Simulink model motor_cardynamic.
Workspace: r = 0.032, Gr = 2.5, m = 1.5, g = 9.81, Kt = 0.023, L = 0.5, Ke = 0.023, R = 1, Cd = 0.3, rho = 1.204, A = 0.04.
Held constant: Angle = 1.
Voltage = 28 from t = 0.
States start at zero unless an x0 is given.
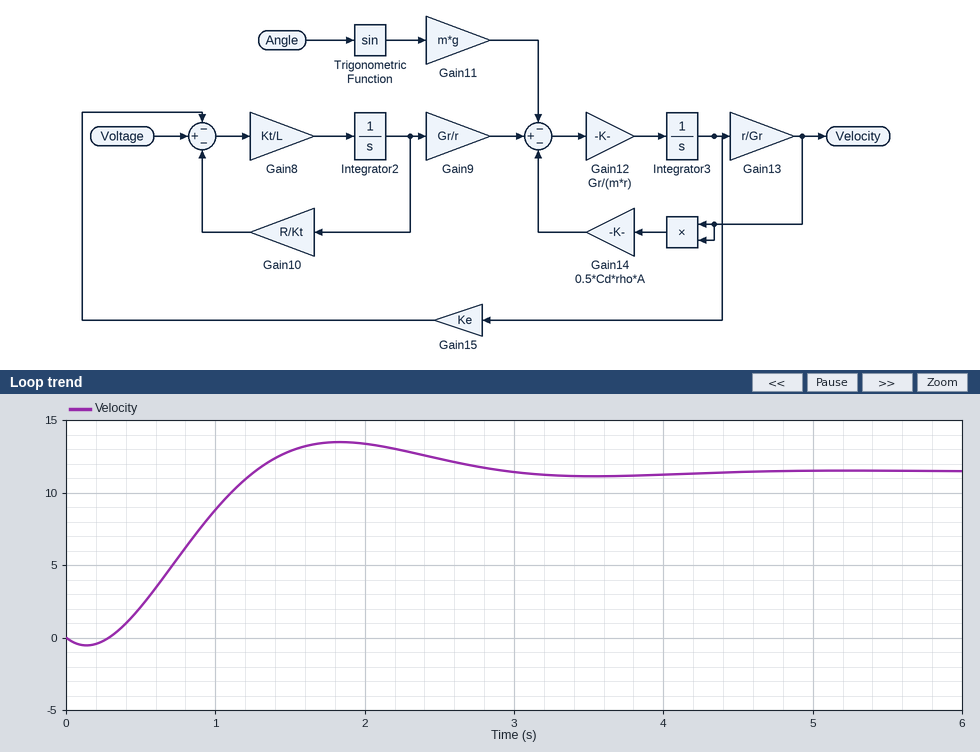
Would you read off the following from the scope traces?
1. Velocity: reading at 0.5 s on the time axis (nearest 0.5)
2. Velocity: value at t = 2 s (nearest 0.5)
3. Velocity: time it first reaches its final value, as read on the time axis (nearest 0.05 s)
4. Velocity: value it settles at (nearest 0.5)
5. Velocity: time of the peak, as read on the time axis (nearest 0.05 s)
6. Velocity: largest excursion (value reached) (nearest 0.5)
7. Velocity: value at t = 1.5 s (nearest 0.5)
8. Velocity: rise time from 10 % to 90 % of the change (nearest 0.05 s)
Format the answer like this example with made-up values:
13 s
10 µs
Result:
2.0
13.5
1.25 s
11.5
1.85 s
13.5
13.0
0.70 s
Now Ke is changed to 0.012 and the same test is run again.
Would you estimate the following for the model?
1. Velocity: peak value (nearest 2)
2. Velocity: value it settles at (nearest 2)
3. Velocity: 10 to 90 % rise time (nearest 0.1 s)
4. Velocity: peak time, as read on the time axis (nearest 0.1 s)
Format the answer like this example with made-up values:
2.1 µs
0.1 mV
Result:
22
20
1.2 s
2.8 s
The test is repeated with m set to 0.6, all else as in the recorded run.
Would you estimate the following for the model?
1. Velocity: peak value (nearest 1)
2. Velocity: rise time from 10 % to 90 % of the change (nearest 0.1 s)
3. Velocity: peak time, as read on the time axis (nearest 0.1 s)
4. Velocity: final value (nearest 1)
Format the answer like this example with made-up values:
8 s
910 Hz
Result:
18
0.4 s
1.0 s
14
